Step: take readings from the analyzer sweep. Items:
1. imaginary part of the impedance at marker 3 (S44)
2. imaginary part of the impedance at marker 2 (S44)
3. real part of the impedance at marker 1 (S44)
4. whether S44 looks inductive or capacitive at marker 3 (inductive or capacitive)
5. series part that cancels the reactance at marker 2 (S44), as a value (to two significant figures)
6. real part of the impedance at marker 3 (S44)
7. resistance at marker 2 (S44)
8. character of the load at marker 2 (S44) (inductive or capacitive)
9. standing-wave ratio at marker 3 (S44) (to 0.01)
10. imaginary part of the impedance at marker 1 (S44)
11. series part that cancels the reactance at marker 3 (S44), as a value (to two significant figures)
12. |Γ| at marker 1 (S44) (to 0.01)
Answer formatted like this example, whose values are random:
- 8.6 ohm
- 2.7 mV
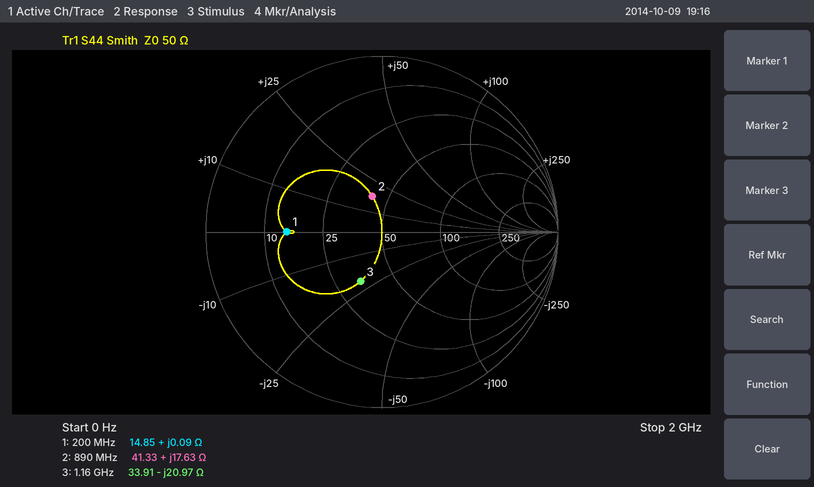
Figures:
- -20.97 Ω
- +17.63 Ω
- 14.85 Ω
- capacitive
- 10 pF
- 33.91 Ω
- 41.33 Ω
- inductive
- 1.88
- +0.09 Ω
- 2.9 nH
- 0.54
